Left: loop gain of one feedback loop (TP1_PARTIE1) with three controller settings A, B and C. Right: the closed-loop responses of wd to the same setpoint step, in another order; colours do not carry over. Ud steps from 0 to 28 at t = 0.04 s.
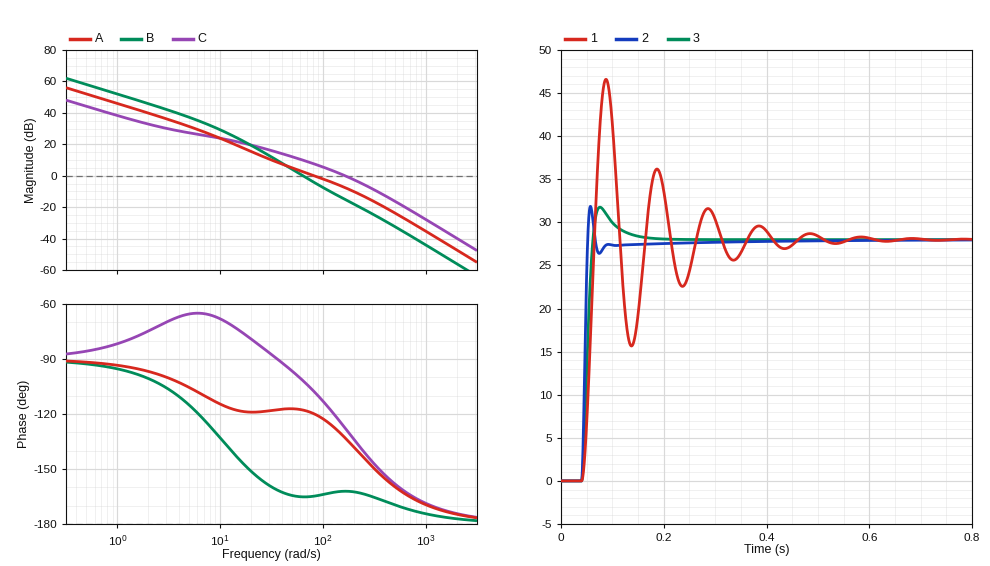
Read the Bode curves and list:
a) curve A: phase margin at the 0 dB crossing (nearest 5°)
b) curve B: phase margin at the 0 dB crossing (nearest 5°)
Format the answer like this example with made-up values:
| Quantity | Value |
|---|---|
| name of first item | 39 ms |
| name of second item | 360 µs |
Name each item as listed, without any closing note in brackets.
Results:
| Quantity | Value |
|---|---|
| curve A: phase margin at the 0 dB crossing | 60° |
| curve B: phase margin at the 0 dB crossing | 15° |
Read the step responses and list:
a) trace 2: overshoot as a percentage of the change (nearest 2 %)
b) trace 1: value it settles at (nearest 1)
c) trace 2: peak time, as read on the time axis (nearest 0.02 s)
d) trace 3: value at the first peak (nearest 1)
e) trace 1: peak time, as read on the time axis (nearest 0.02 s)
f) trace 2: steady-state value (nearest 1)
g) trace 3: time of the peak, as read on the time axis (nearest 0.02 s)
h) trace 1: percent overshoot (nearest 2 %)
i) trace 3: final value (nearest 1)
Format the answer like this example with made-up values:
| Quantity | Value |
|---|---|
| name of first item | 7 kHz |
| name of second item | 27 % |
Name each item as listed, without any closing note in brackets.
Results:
| Quantity | Value |
|---|---|
| trace 2: overshoot as a percentage of the change | 14 % |
| trace 1: value it settles at | 28 |
| trace 2: peak time, as read on the time axis | 0.06 s |
| trace 3: value at the first peak | 32 |
| trace 1: peak time, as read on the time axis | 0.08 s |
| trace 2: steady-state value | 28 |
| trace 3: time of the peak, as read on the time axis | 0.08 s |
| trace 1: percent overshoot | 66 % |
| trace 3: final value | 28 |
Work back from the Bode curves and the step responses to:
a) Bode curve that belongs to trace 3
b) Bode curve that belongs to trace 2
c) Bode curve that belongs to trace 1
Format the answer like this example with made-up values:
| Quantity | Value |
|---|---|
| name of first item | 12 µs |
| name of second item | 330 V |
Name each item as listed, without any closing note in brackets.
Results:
| Quantity | Value |
|---|---|
| Bode curve that belongs to trace 3 | A |
| Bode curve that belongs to trace 2 | C |
| Bode curve that belongs to trace 1 | B |
